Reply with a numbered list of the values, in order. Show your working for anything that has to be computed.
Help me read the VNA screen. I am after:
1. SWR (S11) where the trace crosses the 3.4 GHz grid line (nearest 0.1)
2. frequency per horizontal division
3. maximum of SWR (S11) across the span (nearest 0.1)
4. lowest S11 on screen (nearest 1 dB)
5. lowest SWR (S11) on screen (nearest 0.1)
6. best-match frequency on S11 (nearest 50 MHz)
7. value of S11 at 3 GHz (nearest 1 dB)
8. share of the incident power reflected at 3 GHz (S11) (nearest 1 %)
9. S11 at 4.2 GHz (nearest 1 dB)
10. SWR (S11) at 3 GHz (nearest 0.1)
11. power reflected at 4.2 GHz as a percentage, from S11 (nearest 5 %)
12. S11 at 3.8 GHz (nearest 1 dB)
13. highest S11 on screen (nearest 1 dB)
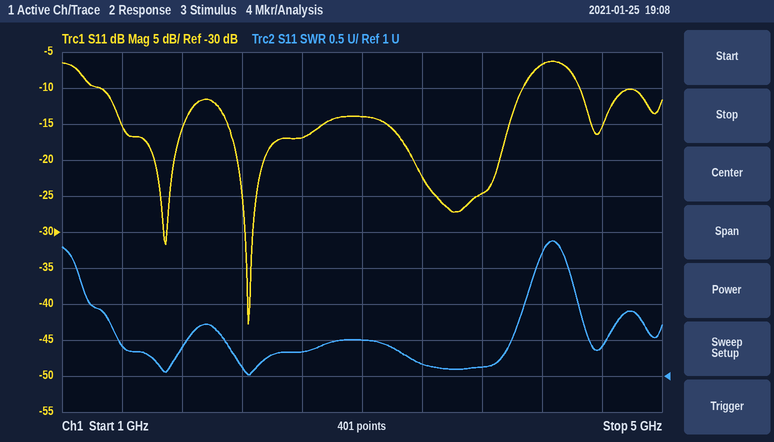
1. 1.2
2. 400 MHz
3. 2.9
4. -43 dB
5. 1.0
6. 2.25 GHz
7. -14 dB
8. 10^(-14/10) ≈ 4 %
9. -7 dB
10. 1.5
11. 10^(-7/10) ≈ 20 %
12. -25 dB
13. -6 dB
